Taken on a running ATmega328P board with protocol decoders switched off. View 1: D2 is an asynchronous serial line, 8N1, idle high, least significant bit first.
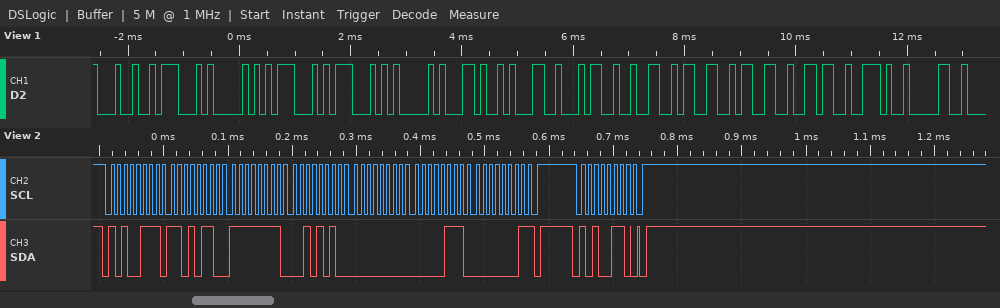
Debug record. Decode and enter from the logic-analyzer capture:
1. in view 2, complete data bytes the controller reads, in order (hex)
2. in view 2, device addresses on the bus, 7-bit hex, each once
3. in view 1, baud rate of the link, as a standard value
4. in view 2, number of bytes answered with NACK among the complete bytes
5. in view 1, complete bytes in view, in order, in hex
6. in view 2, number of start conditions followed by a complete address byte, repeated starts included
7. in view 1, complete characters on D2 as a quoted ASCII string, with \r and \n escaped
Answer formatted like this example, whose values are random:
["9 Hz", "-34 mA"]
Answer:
["D6 FF 2A 00 07 01", "0x53", "9600 baud", "1", "24 47 50 47 47 41 2C 31 34 32 33 33 36 2E 30", "2", "\"$GPGGA,142336.0\""]
